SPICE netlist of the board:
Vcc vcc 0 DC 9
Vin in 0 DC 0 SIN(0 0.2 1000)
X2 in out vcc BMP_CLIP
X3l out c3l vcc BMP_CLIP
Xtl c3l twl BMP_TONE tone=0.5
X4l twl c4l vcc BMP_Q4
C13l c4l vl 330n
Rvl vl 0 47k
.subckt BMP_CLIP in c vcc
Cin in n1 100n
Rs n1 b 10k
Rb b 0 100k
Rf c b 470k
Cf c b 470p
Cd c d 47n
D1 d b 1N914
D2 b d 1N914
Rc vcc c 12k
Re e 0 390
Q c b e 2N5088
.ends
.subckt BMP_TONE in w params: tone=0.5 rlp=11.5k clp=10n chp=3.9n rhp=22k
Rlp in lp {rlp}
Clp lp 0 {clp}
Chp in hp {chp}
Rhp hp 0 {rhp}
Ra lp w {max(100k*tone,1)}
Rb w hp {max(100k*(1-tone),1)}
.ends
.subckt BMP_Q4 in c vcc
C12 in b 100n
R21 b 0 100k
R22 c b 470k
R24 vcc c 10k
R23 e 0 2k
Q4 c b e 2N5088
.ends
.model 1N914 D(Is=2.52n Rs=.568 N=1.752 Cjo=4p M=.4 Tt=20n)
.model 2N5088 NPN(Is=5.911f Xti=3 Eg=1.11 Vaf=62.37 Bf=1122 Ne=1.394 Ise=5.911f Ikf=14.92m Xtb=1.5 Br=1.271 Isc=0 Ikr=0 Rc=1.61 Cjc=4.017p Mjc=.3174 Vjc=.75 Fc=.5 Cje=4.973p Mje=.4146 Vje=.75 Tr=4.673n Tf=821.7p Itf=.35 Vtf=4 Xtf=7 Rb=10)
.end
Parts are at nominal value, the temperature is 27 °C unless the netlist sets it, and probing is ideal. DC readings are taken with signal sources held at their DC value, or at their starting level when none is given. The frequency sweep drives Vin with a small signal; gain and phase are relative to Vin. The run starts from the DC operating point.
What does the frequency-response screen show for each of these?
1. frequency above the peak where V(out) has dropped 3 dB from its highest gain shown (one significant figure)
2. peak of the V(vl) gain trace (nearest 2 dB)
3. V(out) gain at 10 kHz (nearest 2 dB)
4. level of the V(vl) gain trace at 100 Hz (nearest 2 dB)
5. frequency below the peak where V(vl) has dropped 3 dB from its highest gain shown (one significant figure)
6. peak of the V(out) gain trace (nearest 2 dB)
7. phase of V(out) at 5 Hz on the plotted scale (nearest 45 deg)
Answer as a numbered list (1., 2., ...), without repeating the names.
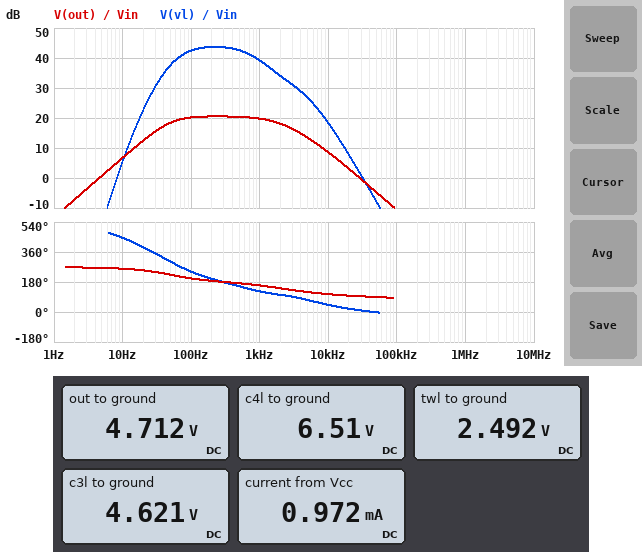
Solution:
1. 2 kHz
2. 44 dB
3. 8 dB
4. 42 dB
5. 70 Hz
6. 20 dB
7. 270 deg
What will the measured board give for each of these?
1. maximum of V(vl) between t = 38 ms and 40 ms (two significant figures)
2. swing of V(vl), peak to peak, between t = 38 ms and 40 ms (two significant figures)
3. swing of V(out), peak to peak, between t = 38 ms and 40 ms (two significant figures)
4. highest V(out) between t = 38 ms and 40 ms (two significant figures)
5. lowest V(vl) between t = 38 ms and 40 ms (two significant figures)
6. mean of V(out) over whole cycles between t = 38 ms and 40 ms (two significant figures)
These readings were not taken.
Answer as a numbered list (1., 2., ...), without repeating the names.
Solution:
1. 540 mV
2. 1.1 V
3. 750 mV
4. 5.1 V
5. -550 mV
6. 4.7 V
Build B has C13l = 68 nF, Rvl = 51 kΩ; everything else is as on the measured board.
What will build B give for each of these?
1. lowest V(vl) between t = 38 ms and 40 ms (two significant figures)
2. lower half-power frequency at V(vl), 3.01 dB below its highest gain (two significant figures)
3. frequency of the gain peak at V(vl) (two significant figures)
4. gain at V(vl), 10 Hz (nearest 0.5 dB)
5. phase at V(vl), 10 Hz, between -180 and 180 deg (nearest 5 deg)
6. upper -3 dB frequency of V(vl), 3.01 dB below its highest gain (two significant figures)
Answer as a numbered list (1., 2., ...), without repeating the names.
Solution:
1. -540 mV
2. 80 Hz
3. 240 Hz
4. -4.5 dB
5. 120 deg
6. 800 Hz
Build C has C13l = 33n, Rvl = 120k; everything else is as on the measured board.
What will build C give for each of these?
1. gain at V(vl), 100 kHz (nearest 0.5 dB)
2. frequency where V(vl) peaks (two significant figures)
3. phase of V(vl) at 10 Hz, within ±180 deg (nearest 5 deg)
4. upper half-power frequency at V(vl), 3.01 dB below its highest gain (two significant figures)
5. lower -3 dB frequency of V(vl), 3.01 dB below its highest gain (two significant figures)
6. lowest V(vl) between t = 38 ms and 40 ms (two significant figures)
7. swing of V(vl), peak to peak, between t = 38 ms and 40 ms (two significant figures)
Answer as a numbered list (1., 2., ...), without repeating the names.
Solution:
1. -19.0 dB
2. 240 Hz
3. 120 deg
4. 800 Hz
5. 80 Hz
6. -590 mV
7. 1.2 V
